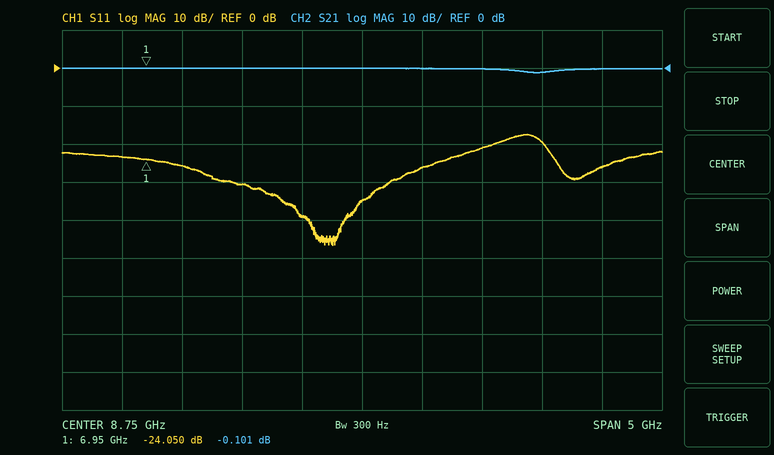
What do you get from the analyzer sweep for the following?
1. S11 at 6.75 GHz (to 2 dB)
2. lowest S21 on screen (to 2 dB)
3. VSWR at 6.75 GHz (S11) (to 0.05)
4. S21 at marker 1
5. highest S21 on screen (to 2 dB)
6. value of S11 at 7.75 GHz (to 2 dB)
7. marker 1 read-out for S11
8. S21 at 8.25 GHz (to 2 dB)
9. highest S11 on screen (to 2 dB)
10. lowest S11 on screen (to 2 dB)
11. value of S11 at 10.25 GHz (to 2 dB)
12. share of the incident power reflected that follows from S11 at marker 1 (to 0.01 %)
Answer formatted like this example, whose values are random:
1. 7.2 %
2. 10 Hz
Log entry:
1. -24 dB
2. -2 dB
3. 1.15
4. -0.101 dB
5. 0 dB
6. -30 dB
7. -24.050 dB
8. 0 dB
9. -18 dB
10. -46 dB
11. -20 dB
12. 0.39 %
